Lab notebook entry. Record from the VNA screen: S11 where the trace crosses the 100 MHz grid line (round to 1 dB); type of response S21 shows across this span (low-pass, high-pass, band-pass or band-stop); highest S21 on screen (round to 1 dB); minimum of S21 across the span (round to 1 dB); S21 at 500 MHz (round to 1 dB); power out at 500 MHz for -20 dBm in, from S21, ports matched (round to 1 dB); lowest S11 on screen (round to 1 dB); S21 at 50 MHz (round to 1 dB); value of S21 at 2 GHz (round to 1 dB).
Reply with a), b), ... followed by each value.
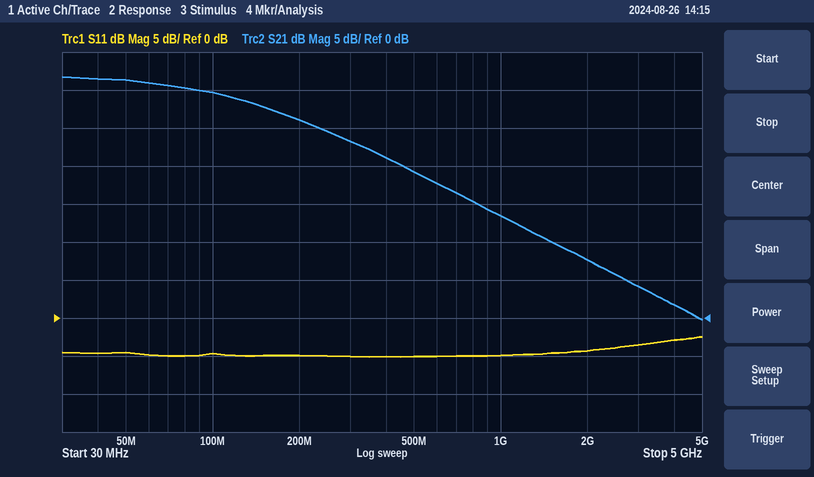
a) -5 dB
b) low-pass
c) 32 dB
d) 0 dB
e) 19 dB
f) -1 dBm
g) -5 dB
h) 31 dB
i) 8 dB
